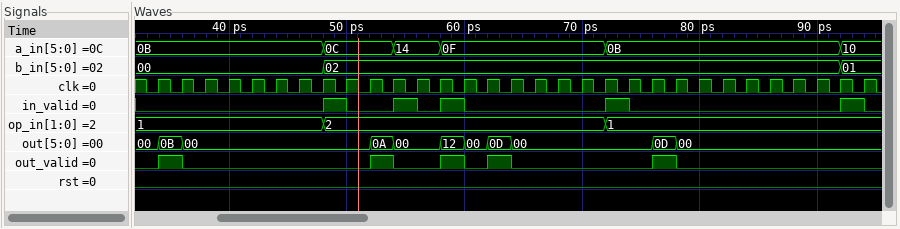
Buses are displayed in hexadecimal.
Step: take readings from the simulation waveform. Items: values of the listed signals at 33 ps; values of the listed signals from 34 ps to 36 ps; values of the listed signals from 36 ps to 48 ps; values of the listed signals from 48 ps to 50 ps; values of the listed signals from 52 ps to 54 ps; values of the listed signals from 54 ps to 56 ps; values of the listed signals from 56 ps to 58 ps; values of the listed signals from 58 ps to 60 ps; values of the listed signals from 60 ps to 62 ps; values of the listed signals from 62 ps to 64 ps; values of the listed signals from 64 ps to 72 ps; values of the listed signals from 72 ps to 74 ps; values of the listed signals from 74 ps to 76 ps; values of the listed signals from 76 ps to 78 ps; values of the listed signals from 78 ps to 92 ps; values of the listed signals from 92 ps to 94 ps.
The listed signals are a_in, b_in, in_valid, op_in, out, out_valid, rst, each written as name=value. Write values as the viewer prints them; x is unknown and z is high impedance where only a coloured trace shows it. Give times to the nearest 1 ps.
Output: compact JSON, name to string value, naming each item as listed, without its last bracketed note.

{"values of the listed signals at 33 ps": "a_in=0B, b_in=00, in_valid=0, op_in=1, out=00, out_valid=0, rst=0", "values of the listed signals from 34 ps to 36 ps": "a_in=0B, b_in=00, in_valid=0, op_in=1, out=0B, out_valid=1, rst=0", "values of the listed signals from 36 ps to 48 ps": "a_in=0B, b_in=00, in_valid=0, op_in=1, out=00, out_valid=0, rst=0", "values of the listed signals from 48 ps to 50 ps": "a_in=0C, b_in=02, in_valid=1, op_in=2, out=00, out_valid=0, rst=0", "values of the listed signals from 52 ps to 54 ps": "a_in=0C, b_in=02, in_valid=0, op_in=2, out=0A, out_valid=1, rst=0", "values of the listed signals from 54 ps to 56 ps": "a_in=14, b_in=02, in_valid=1, op_in=2, out=00, out_valid=0, rst=0", "values of the listed signals from 56 ps to 58 ps": "a_in=14, b_in=02, in_valid=0, op_in=2, out=00, out_valid=0, rst=0", "values of the listed signals from 58 ps to 60 ps": "a_in=0F, b_in=02, in_valid=1, op_in=2, out=12, out_valid=1, rst=0", "values of the listed signals from 60 ps to 62 ps": "a_in=0F, b_in=02, in_valid=0, op_in=2, out=00, out_valid=0, rst=0", "values of the listed signals from 62 ps to 64 ps": "a_in=0F, b_in=02, in_valid=0, op_in=2, out=0D, out_valid=1, rst=0", "values of the listed signals from 64 ps to 72 ps": "a_in=0F, b_in=02, in_valid=0, op_in=2, out=00, out_valid=0, rst=0", "values of the listed signals from 72 ps to 74 ps": "a_in=0B, b_in=02, in_valid=1, op_in=1, out=00, out_valid=0, rst=0", "values of the listed signals from 74 ps to 76 ps": "a_in=0B, b_in=02, in_valid=0, op_in=1, out=00, out_valid=0, rst=0", "values of the listed signals from 76 ps to 78 ps": "a_in=0B, b_in=02, in_valid=0, op_in=1, out=0D, out_valid=1, rst=0", "values of the listed signals from 78 ps to 92 ps": "a_in=0B, b_in=02, in_valid=0, op_in=1, out=00, out_valid=0, rst=0", "values of the listed signals from 92 ps to 94 ps": "a_in=10, b_in=01, in_valid=1, op_in=1, out=00, out_valid=0, rst=0"}
